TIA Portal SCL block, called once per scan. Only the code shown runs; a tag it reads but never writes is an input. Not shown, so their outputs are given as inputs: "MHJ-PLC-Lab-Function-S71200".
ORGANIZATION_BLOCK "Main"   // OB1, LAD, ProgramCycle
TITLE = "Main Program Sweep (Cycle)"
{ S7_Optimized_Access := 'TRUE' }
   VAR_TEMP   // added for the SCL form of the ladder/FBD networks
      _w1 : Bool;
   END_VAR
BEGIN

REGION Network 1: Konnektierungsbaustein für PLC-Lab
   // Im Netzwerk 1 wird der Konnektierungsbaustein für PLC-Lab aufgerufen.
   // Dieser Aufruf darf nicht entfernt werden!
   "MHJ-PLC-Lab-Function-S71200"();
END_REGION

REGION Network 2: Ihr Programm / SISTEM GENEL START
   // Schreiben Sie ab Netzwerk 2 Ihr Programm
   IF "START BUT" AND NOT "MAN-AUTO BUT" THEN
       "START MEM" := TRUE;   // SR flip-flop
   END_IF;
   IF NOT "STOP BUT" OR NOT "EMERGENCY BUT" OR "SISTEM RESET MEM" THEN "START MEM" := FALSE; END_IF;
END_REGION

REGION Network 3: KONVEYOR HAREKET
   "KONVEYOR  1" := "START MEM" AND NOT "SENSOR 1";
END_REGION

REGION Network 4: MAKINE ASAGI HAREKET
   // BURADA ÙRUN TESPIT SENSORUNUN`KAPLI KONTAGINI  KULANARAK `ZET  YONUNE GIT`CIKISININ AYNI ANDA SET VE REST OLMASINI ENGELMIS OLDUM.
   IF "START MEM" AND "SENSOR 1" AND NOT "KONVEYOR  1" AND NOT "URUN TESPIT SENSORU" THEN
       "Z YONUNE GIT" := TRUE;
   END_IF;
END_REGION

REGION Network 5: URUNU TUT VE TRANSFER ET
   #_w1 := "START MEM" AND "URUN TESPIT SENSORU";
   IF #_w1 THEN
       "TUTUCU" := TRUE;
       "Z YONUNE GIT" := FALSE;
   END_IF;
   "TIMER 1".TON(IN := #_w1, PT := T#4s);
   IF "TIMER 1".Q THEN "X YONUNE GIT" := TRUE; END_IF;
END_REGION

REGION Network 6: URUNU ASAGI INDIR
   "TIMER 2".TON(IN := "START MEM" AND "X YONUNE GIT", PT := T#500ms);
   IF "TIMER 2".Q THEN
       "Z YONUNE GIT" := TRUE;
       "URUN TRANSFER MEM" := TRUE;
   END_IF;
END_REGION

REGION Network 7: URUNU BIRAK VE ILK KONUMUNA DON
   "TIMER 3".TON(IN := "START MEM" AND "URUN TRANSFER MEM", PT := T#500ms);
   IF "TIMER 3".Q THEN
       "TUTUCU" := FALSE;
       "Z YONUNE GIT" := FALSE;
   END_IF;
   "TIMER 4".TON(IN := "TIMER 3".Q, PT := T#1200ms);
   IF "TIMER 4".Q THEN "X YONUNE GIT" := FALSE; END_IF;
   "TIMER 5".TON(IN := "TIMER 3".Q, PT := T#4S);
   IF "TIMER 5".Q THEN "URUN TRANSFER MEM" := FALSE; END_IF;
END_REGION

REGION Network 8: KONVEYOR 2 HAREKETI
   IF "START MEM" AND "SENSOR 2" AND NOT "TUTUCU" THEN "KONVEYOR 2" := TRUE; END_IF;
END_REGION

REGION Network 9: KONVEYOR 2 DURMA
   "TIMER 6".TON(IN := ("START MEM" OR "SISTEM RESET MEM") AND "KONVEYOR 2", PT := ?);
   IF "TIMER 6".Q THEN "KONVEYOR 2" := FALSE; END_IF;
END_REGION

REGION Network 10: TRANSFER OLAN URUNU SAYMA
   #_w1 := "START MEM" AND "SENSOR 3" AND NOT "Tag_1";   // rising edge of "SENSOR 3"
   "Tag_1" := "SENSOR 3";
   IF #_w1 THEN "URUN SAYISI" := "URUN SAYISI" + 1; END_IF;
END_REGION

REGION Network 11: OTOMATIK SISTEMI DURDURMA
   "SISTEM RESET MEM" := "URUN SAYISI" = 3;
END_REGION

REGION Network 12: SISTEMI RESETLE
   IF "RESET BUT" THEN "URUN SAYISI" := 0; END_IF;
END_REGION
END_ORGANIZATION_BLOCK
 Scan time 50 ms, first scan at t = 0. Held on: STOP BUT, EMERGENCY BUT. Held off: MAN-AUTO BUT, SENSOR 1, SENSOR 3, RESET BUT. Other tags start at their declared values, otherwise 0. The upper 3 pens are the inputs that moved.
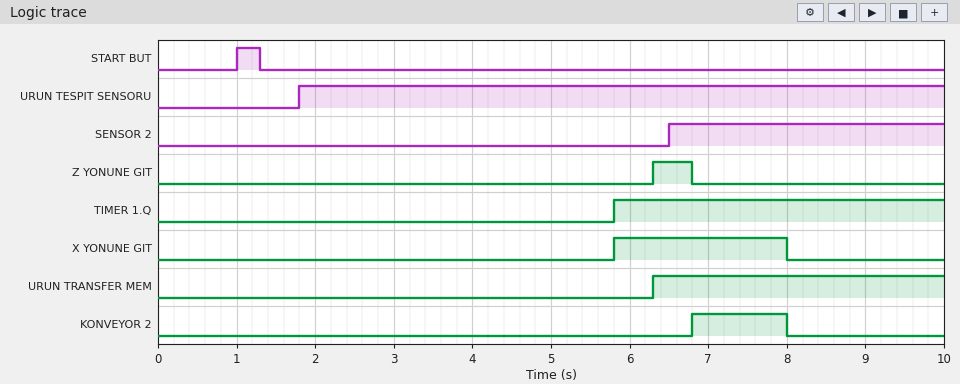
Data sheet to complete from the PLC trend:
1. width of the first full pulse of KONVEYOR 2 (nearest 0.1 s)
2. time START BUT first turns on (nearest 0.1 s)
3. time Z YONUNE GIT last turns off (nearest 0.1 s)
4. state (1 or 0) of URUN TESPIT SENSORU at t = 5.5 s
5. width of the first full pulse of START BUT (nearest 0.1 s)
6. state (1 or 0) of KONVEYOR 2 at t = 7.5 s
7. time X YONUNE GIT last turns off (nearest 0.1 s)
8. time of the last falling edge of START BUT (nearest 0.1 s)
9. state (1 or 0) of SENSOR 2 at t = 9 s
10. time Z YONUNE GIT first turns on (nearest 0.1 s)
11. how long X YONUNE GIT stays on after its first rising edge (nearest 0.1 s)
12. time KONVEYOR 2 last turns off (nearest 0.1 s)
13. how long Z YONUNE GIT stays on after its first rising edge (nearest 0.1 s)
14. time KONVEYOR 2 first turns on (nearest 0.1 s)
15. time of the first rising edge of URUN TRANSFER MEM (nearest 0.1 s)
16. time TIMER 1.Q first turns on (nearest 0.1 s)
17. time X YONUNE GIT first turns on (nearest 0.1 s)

1.2 s
1.0 s
6.8 s
1
0.3 s
1
8.0 s
1.3 s
1
6.3 s
2.2 s
8.0 s
0.5 s
6.8 s
6.3 s
5.8 s
5.8 s
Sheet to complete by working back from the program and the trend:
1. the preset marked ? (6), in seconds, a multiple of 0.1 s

1.2 s
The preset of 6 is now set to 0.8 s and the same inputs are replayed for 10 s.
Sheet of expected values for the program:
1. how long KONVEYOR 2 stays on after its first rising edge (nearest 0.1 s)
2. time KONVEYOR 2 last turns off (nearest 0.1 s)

0.8 s
7.6 s
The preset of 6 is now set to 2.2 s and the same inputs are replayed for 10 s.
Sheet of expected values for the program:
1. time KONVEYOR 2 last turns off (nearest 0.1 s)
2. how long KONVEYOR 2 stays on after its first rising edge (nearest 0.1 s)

9.0 s
2.2 s
